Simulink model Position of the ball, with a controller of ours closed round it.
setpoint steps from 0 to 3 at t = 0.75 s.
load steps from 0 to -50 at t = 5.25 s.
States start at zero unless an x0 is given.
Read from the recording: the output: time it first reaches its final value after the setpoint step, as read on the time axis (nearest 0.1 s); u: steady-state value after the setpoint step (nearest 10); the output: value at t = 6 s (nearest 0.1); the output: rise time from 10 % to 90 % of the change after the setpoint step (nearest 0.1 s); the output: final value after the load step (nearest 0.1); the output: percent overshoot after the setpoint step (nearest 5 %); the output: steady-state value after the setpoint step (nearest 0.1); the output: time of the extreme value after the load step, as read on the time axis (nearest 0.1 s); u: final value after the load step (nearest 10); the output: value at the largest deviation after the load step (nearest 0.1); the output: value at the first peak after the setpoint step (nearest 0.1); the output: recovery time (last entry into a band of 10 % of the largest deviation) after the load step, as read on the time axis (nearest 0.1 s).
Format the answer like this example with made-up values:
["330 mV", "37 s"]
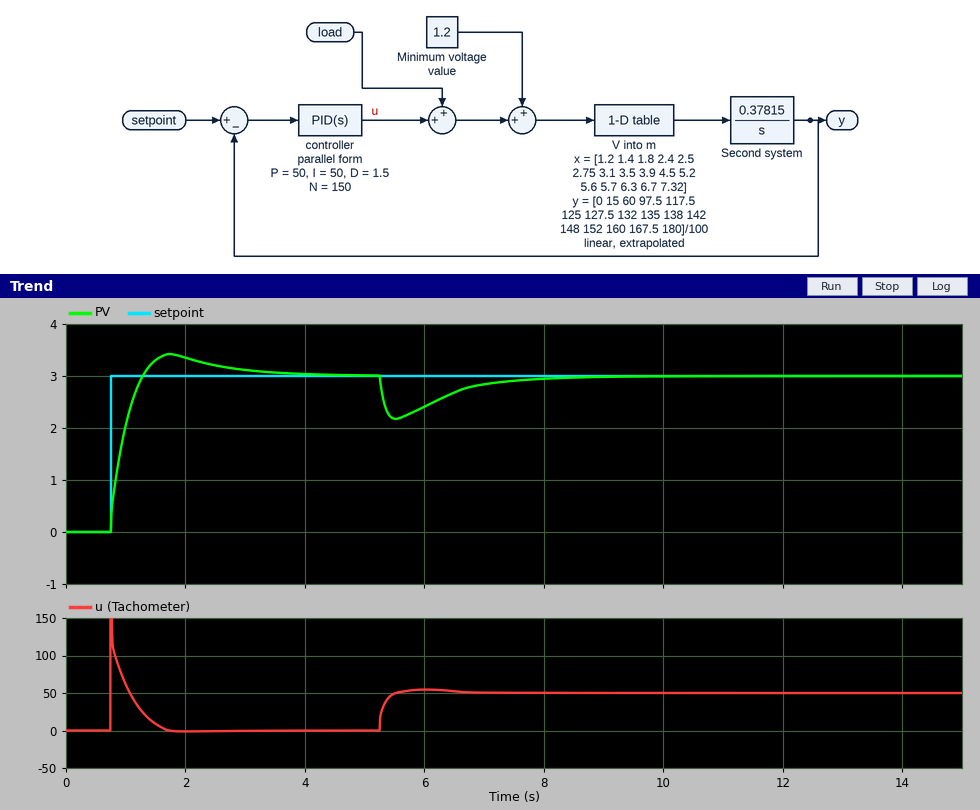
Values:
["1.3 s", "0", "2.4", "0.4 s", "3.0", "15 %", "3.0", "5.5 s", "50", "2.2", "3.4", "7.6 s"]
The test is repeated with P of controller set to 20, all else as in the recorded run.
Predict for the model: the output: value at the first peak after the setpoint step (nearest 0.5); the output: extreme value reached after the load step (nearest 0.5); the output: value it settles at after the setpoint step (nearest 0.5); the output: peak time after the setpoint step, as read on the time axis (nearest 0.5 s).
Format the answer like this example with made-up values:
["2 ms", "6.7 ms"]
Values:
["4.0", "1.5", "3.0", "2.0 s"]
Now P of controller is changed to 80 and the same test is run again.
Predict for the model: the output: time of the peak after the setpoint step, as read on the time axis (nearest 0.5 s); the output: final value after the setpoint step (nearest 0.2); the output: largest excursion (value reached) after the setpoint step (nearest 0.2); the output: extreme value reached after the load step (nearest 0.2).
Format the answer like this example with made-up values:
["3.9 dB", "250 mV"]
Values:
["1.5 s", "3.0", "3.2", "2.4"]
